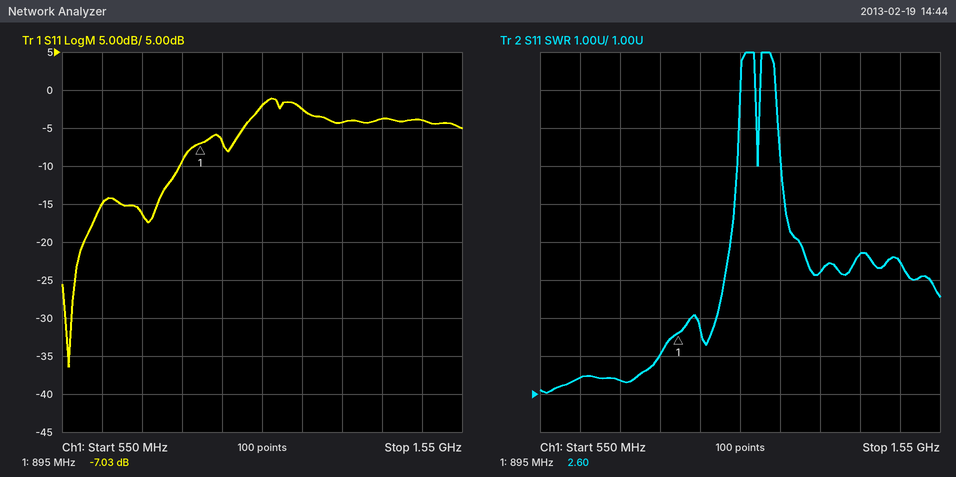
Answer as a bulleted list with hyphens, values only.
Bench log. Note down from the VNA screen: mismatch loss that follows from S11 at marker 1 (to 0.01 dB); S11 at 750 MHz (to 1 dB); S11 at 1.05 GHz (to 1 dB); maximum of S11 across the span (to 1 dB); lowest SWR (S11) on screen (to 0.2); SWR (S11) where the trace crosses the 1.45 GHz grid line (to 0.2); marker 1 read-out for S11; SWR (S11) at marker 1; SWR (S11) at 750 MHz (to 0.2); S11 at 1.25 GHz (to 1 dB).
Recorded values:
- 0.96 dB
- -16 dB
- -2 dB
- -1 dB
- 1.0
- 4.4
- -7.03 dB
- 2.60
- 1.4
- -4 dB
